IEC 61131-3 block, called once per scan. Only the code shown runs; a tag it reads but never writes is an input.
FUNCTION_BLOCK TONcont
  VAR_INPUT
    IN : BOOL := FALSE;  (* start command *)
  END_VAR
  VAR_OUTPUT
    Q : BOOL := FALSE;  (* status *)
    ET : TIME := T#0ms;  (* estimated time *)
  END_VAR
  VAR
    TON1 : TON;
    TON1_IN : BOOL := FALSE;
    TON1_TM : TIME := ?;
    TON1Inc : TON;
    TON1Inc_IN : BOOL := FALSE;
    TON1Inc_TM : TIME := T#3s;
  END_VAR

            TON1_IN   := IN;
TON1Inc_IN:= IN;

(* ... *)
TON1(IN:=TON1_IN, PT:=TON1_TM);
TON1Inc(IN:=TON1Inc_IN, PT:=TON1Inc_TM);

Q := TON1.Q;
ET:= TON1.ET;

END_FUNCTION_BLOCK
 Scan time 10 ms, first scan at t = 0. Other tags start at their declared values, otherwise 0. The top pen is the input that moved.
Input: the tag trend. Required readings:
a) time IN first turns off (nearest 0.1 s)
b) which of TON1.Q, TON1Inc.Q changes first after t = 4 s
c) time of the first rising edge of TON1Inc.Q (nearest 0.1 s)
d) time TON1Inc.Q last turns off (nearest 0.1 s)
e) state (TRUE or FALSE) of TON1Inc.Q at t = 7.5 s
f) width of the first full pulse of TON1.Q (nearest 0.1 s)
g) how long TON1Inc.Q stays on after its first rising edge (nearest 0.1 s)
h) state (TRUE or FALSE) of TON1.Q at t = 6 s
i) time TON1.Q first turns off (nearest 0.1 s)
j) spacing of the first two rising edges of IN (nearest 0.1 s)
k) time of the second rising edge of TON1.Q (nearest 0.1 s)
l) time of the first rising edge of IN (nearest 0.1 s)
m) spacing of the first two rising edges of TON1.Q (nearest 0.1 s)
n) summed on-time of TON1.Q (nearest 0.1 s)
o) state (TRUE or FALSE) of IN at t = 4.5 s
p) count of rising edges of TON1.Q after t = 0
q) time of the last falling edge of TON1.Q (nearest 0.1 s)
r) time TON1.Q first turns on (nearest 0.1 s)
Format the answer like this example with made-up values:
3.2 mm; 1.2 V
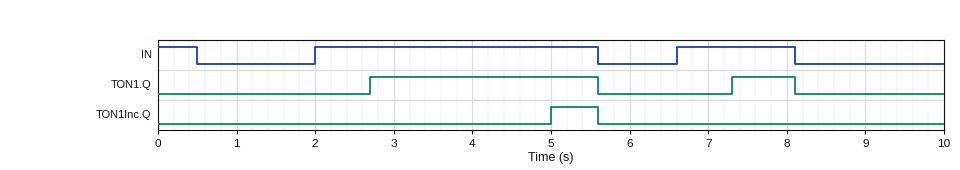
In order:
0.5 s; TON1Inc.Q; 5.0 s; 5.6 s; FALSE; 2.9 s; 0.6 s; FALSE; 5.6 s; 4.6 s; 7.3 s; 2.0 s; 4.6 s; 3.7 s; TRUE; 2; 8.1 s; 2.7 s
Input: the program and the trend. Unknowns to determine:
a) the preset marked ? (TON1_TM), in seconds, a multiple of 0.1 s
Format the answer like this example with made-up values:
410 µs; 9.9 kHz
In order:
0.7 s
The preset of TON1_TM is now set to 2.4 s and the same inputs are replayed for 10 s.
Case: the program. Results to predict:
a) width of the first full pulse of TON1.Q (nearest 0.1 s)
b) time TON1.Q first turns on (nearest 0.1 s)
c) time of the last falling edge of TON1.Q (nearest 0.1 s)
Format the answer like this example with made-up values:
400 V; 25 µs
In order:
1.2 s; 4.4 s; 5.6 s
